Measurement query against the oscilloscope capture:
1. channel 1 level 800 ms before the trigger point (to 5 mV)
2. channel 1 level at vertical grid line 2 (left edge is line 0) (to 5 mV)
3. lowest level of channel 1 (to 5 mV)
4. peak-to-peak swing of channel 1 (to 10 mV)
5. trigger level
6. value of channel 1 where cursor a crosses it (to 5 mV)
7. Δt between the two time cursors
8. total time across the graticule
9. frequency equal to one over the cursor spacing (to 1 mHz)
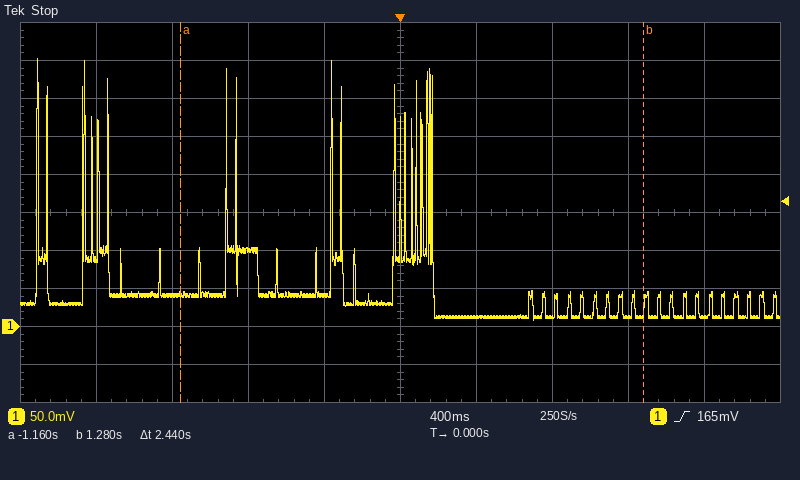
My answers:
100 mV
40 mV
10 mV
340 mV
165 mV
40 mV
2.44 s
4 s
410 mHz
